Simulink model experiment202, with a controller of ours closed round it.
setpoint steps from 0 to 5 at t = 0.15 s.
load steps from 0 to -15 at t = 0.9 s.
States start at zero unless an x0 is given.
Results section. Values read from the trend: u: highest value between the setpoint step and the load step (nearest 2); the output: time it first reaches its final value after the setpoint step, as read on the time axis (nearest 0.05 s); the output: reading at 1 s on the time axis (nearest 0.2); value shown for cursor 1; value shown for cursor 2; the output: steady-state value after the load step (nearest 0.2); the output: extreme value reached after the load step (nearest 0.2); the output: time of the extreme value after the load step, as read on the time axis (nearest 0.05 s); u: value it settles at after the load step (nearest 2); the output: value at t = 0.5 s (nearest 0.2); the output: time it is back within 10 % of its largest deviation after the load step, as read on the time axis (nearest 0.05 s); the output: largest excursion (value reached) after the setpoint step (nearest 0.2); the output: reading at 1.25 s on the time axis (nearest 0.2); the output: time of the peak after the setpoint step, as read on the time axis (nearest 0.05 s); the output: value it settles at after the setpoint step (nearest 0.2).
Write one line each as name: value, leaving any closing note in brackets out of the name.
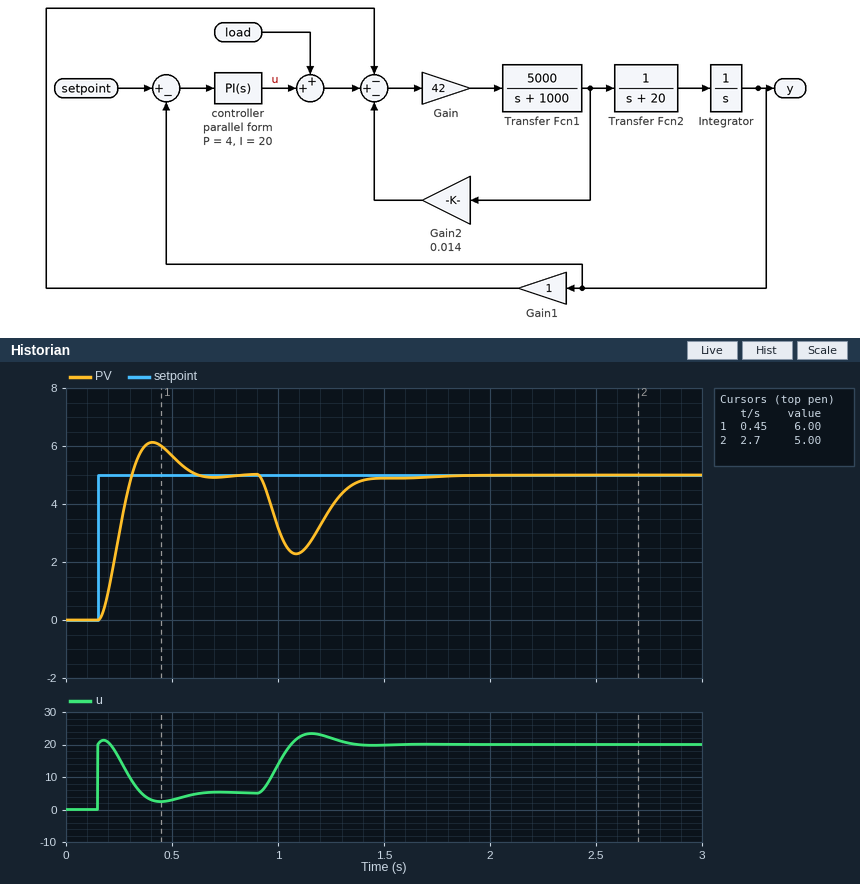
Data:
u: highest value between the setpoint step and the load step: 22
the output: time it first reaches its final value after the setpoint step, as read on the time axis: 0.30 s
the output: reading at 1 s on the time axis: 3.2
value shown for cursor 1: 6.00
value shown for cursor 2: 5.00
the output: steady-state value after the load step: 5.0
the output: extreme value reached after the load step: 2.2
the output: time of the extreme value after the load step, as read on the time axis: 1.10 s
u: value it settles at after the load step: 20
the output: value at t = 0.5 s: 5.6
the output: time it is back within 10 % of its largest deviation after the load step, as read on the time axis: 1.35 s
the output: largest excursion (value reached) after the setpoint step: 6.2
the output: reading at 1.25 s on the time axis: 3.8
the output: time of the peak after the setpoint step, as read on the time axis: 0.40 s
the output: value it settles at after the setpoint step: 5.0
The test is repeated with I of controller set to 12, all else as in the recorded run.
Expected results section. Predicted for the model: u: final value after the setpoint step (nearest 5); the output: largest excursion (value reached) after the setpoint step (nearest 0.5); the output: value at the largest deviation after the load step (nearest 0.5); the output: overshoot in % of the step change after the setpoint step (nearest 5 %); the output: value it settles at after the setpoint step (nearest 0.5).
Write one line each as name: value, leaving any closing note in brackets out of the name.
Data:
u: final value after the setpoint step: 5
the output: largest excursion (value reached) after the setpoint step: 5.5
the output: value at the largest deviation after the load step: 2.0
the output: overshoot in % of the step change after the setpoint step: 10 %
the output: value it settles at after the setpoint step: 5.0
